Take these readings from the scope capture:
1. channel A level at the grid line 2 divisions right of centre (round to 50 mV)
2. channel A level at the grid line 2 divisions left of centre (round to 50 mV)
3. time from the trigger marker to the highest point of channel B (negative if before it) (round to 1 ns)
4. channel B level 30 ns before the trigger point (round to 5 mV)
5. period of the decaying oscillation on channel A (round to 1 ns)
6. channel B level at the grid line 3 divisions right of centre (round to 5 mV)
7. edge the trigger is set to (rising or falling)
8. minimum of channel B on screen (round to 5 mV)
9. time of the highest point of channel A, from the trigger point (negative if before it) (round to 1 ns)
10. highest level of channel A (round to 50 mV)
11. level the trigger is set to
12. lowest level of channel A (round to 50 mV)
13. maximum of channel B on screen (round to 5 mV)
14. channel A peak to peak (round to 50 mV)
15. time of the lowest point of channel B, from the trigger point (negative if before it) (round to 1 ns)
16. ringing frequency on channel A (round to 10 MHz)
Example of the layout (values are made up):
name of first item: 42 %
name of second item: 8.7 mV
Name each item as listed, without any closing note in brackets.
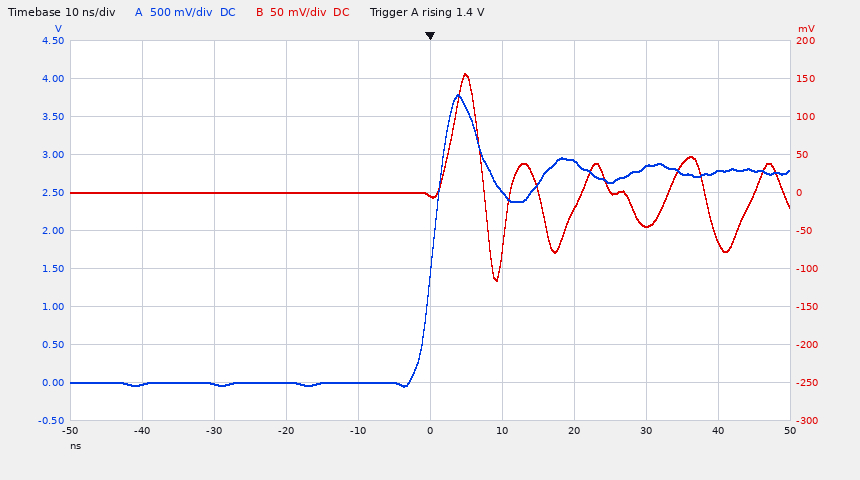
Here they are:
channel A level at the grid line 2 divisions right of centre: 2.90 V
channel A level at the grid line 2 divisions left of centre: 0 mV
time from the trigger marker to the highest point of channel B (negative if before it): +5 ns
channel B level 30 ns before the trigger point: 0 mV
period of the decaying oscillation on channel A: 14 ns
channel B level at the grid line 3 divisions right of centre: -45 mV
edge the trigger is set to: rising
minimum of channel B on screen: -115 mV
time of the highest point of channel A, from the trigger point (negative if before it): +4 ns
highest level of channel A: 3.80 V
level the trigger is set to: 1.4 V
lowest level of channel A: -50 mV
maximum of channel B on screen: 155 mV
channel A peak to peak: 3.85 V
time of the lowest point of channel B, from the trigger point (negative if before it): +9 ns
ringing frequency on channel A: 70 MHz
